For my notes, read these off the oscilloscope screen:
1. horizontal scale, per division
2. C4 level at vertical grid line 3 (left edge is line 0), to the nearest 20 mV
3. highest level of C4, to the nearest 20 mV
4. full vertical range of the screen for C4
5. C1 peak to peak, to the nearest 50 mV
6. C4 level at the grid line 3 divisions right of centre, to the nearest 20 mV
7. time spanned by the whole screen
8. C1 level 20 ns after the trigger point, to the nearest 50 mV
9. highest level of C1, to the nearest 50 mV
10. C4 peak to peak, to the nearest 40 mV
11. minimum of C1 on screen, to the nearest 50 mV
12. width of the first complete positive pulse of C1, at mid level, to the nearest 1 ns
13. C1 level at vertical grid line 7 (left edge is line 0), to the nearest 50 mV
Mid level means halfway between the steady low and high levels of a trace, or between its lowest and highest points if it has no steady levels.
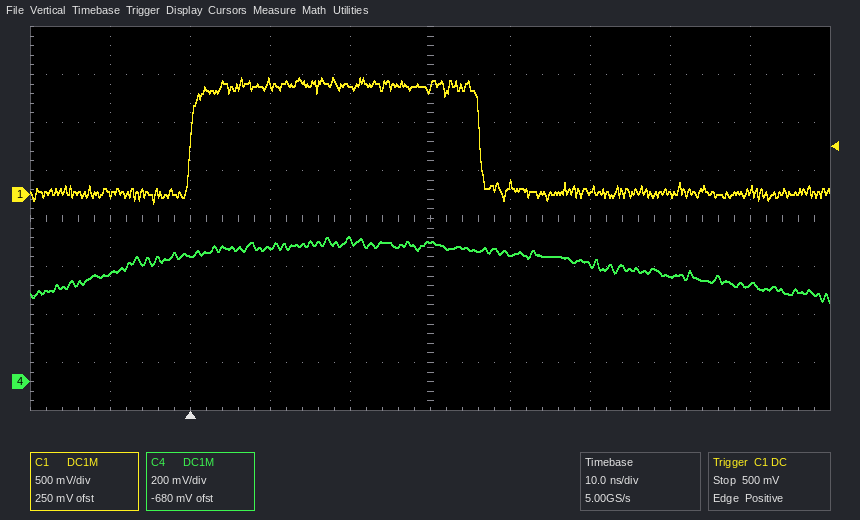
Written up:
10 ns
560 mV
600 mV
1.6 V
1.30 V
440 mV
100 ns
1.10 V
1.20 V
280 mV
-100 mV
36 ns
50 mV
